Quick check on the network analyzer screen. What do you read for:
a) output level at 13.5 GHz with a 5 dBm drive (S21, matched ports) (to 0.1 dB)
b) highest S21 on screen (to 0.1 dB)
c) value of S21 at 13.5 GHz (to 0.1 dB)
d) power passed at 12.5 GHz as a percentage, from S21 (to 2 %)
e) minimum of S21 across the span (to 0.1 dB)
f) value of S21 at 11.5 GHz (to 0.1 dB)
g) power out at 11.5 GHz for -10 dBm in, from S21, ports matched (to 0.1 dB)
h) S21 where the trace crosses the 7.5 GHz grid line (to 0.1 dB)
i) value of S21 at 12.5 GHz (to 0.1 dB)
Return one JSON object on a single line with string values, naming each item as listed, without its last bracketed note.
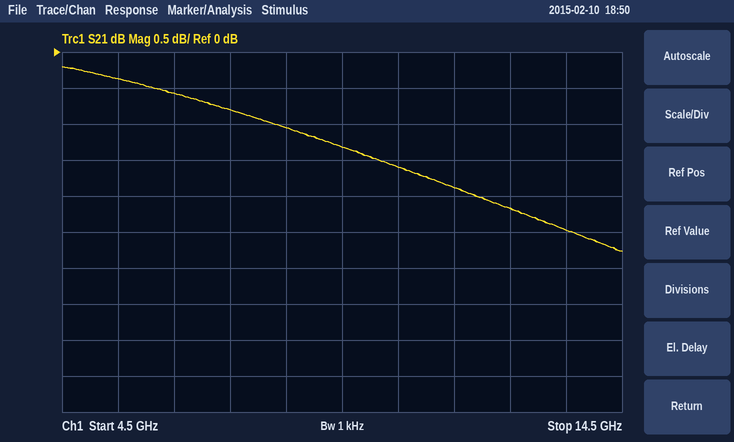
{"output level at 13.5 GHz with a 5 dBm drive (S21, matched ports)": "2.5 dBm", "highest S21 on screen": "-0.2 dB", "value of S21 at 13.5 GHz": "-2.5 dB", "power passed at 12.5 GHz as a percentage, from S21": "60 %", "minimum of S21 across the span": "-2.8 dB", "value of S21 at 11.5 GHz": "-1.9 dB", "power out at 11.5 GHz for -10 dBm in, from S21, ports matched": "-11.9 dBm", "S21 where the trace crosses the 7.5 GHz grid line": "-0.8 dB", "value of S21 at 12.5 GHz": "-2.2 dB"}
